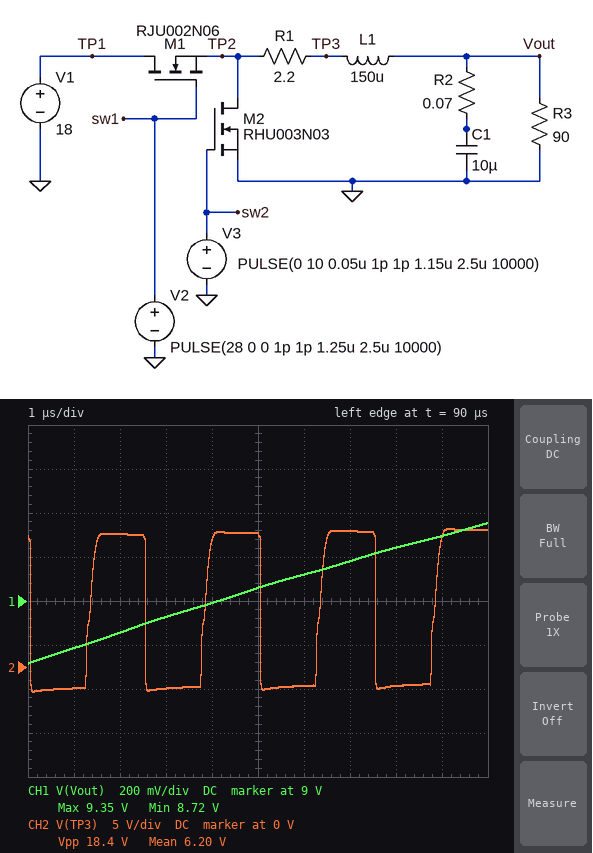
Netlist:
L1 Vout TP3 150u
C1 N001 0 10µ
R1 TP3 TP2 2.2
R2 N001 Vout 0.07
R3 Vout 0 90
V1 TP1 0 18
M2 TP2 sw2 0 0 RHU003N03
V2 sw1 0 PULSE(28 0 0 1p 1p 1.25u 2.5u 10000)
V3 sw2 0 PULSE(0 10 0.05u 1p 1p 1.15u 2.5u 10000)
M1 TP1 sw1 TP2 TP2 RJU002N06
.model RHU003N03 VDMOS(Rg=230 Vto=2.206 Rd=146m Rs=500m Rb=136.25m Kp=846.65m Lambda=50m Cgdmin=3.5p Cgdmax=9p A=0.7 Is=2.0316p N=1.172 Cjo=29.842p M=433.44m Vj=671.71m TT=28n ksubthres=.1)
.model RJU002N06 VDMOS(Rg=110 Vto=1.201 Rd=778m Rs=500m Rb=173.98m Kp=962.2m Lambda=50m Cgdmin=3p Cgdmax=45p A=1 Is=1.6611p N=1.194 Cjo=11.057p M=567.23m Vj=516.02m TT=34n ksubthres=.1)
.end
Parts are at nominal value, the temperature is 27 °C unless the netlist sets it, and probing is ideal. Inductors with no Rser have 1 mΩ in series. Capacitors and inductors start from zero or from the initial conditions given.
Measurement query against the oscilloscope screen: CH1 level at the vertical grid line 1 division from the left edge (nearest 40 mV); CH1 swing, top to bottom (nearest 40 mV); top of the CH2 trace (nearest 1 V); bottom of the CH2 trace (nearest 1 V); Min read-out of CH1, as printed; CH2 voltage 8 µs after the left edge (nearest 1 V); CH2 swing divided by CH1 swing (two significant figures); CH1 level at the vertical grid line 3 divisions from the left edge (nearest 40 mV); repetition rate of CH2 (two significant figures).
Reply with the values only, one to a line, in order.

8.80 V
640 mV
16 V
-3 V
8.72 V
-2 V
29
8.92 V
400 kHz
